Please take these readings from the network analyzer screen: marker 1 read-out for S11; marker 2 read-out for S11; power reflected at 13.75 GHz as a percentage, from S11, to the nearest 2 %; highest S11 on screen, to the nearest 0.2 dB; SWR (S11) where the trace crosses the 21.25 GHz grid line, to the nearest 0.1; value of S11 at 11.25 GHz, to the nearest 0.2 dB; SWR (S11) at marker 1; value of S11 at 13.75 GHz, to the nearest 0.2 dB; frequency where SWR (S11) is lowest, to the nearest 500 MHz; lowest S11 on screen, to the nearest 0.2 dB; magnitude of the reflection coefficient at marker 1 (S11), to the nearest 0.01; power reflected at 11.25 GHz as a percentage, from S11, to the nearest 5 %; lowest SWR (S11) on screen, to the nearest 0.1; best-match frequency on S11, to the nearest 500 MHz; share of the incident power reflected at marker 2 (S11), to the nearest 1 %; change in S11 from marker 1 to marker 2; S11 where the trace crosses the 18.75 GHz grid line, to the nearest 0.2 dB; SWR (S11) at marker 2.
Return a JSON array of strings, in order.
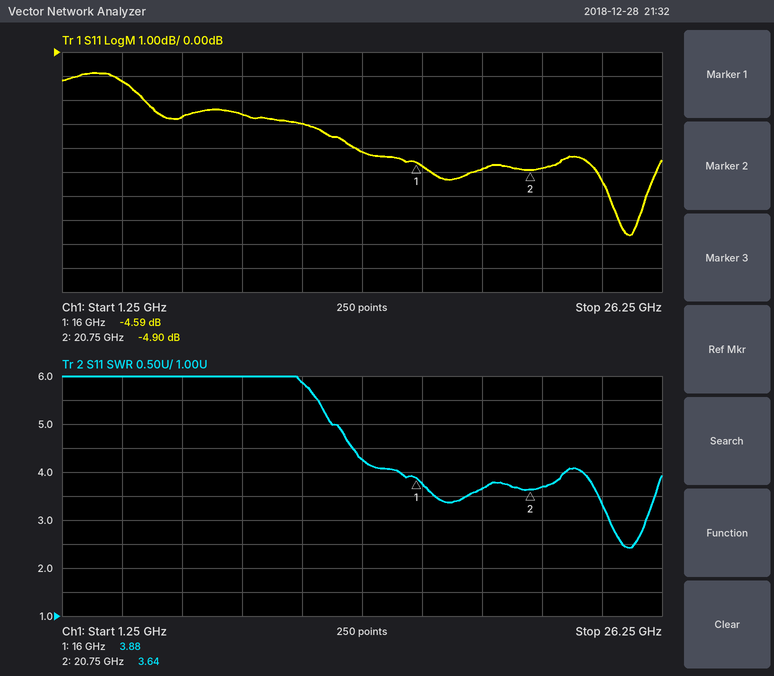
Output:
["-4.59 dB", "-4.90 dB", "38 %", "-0.8 dB", "3.7", "-3.0 dB", "3.88", "-4.2 dB", "25.0 GHz", "-7.6 dB", "0.59", "50 %", "2.4", "25.0 GHz", "32 %", "-0.31 dB", "-4.8 dB", "3.64"]
